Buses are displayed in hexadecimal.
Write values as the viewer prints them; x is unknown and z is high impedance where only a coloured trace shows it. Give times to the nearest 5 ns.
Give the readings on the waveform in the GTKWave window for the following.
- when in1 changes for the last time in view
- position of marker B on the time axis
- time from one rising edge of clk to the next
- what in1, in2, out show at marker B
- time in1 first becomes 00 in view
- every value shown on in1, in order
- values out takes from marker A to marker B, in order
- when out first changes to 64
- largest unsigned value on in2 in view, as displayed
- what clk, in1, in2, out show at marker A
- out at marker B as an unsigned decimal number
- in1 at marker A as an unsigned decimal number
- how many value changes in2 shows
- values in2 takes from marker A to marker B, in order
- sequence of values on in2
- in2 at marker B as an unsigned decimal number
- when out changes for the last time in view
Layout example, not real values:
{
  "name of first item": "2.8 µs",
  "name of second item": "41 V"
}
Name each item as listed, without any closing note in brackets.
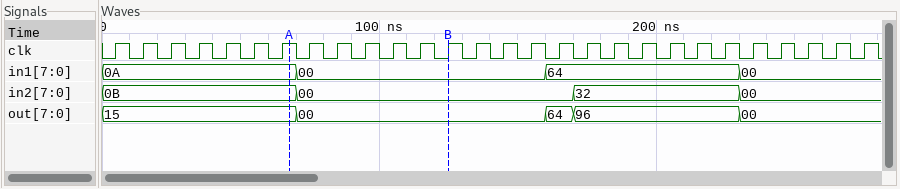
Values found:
{
  "when in1 changes for the last time in view": "230 ns",
  "position of marker B on the time axis": "125 ns",
  "time from one rising edge of clk to the next": "10 ns",
  "what in1, in2, out show at marker B": "in1=00, in2=00, out=00",
  "time in1 first becomes 00 in view": "70 ns",
  "every value shown on in1, in order": "0A, 00, 64, 00",
  "values out takes from marker A to marker B, in order": "15, 00",
  "when out first changes to 64": "160 ns",
  "largest unsigned value on in2 in view, as displayed": "32",
  "what clk, in1, in2, out show at marker A": "clk=1, in1=0A, in2=0B, out=15",
  "out at marker B as an unsigned decimal number": "0",
  "in1 at marker A as an unsigned decimal number": "10",
  "how many value changes in2 shows": "3",
  "values in2 takes from marker A to marker B, in order": "0B, 00",
  "sequence of values on in2": "0B, 00, 32, 00",
  "in2 at marker B as an unsigned decimal number": "0",
  "when out changes for the last time in view": "230 ns"
}
